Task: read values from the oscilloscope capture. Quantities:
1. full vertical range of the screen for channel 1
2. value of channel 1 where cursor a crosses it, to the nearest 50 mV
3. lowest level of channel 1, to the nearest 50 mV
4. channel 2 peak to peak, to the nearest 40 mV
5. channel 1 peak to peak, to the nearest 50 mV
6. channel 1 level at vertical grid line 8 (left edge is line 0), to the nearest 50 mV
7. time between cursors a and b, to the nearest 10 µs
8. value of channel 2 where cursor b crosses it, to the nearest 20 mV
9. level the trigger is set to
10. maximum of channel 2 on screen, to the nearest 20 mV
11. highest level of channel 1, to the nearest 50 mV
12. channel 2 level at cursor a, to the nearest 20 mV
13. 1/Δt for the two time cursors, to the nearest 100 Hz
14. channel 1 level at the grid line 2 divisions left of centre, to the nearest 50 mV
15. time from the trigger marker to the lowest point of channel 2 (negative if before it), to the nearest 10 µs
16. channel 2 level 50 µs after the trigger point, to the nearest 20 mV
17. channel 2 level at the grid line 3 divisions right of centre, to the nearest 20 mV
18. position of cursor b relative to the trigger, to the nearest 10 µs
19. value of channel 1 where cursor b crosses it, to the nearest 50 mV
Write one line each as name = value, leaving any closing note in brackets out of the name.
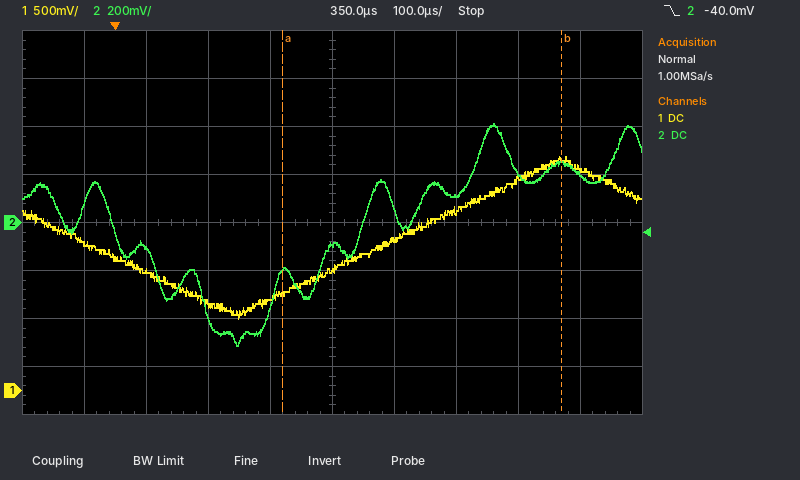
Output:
full vertical range of the screen for channel 1 = 4 V
value of channel 1 where cursor a crosses it, to the nearest 50 mV = 1.00 V
lowest level of channel 1, to the nearest 50 mV = 750 mV
channel 2 peak to peak, to the nearest 40 mV = 920 mV
channel 1 peak to peak, to the nearest 50 mV = 1.70 V
channel 1 level at vertical grid line 8 (left edge is line 0), to the nearest 50 mV = 2.20 V
time between cursors a and b, to the nearest 10 µs = 450 µs
value of channel 2 where cursor b crosses it, to the nearest 20 mV = 240 mV
level the trigger is set to = -40.0 mV
maximum of channel 2 on screen, to the nearest 20 mV = 420 mV
highest level of channel 1, to the nearest 50 mV = 2.45 V
channel 2 level at cursor a, to the nearest 20 mV = -200 mV
1/Δt for the two time cursors, to the nearest 100 Hz = 2.2 kHz
channel 1 level at the grid line 2 divisions left of centre, to the nearest 50 mV = 900 mV
time from the trigger marker to the lowest point of channel 2 (negative if before it), to the nearest 10 µs = +200 µs
channel 2 level 50 µs after the trigger point, to the nearest 20 mV = -100 mV
channel 2 level at the grid line 3 divisions right of centre, to the nearest 20 mV = 200 mV
position of cursor b relative to the trigger, to the nearest 10 µs = +720 µs
value of channel 1 where cursor b crosses it, to the nearest 50 mV = 2.40 V
